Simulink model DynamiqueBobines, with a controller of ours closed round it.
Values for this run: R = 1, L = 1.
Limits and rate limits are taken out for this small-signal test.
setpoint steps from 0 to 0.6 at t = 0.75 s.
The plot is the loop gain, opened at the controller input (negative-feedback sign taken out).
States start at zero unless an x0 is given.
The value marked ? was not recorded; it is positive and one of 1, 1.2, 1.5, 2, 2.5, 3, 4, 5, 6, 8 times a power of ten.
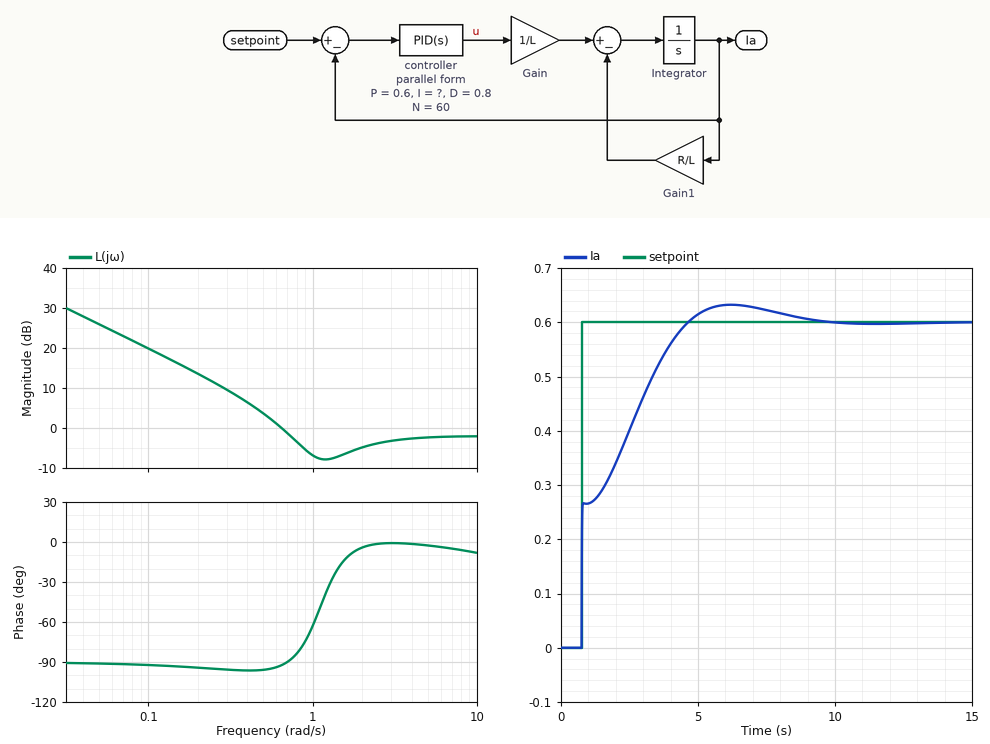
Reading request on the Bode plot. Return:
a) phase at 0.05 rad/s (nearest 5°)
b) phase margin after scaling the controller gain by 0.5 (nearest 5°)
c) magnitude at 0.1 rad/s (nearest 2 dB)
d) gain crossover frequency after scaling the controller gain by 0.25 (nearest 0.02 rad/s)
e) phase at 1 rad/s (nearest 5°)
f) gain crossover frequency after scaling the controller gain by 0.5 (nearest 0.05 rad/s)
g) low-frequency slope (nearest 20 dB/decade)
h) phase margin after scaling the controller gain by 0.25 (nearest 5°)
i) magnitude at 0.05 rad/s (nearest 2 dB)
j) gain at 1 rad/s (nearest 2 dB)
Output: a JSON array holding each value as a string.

["-90°", "85°", "20 dB", "0.24 rad/s", "-65°", "0.40 rad/s", "-20 dB/decade", "85°", "26 dB", "-6 dB"]
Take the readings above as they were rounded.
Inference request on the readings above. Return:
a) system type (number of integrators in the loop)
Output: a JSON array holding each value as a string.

["1"]
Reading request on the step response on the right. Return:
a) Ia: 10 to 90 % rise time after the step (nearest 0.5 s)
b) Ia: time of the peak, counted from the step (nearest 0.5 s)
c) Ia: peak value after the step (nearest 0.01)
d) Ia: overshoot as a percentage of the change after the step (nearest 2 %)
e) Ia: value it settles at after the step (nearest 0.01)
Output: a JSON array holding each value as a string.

["3.0 s", "5.5 s", "0.63", "6 %", "0.60"]
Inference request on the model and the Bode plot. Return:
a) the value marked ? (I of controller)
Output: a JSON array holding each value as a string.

["1"]
